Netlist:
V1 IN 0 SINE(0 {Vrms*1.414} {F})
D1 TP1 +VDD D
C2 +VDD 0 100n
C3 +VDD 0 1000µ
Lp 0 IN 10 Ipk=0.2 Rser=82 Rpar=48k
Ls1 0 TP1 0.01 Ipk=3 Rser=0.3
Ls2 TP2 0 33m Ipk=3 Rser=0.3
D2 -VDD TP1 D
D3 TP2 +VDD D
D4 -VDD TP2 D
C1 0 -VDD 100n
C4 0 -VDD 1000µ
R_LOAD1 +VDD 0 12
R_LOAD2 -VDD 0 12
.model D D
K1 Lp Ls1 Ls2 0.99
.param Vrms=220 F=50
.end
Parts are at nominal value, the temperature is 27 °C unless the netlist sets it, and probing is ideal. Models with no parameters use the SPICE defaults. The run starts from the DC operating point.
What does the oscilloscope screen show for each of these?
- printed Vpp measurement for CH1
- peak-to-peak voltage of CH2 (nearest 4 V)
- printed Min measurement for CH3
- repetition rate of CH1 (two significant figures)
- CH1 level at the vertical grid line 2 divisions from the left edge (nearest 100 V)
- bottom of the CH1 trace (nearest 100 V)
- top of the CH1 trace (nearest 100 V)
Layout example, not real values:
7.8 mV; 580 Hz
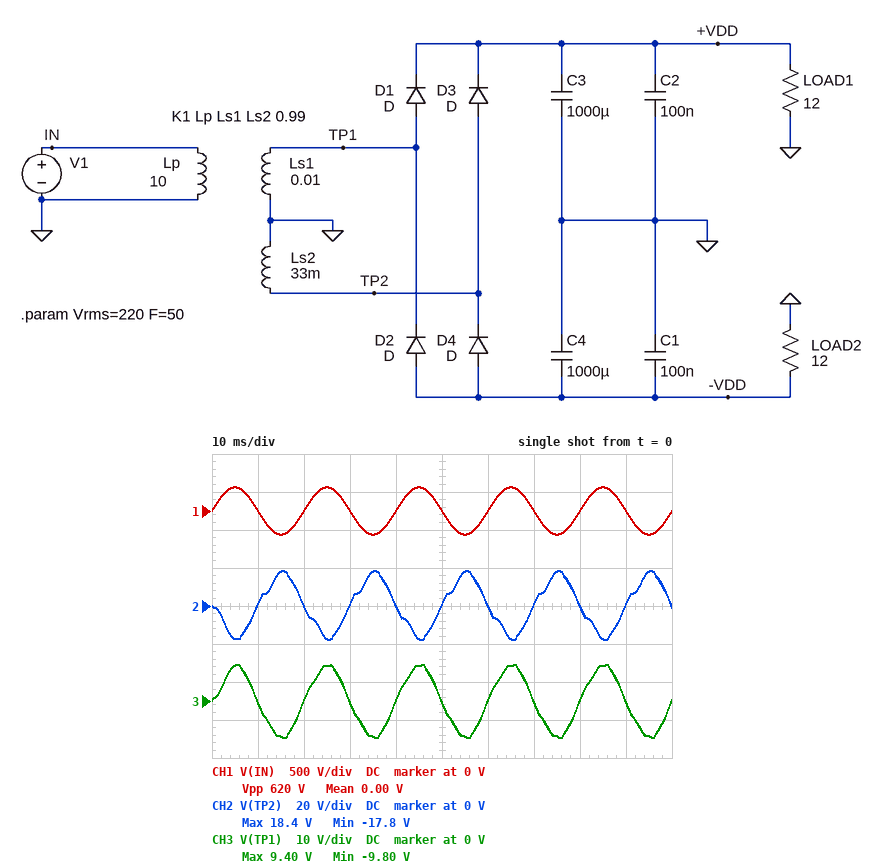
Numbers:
620 V; 36 V; -9.80 V; 50 Hz; 0 V; -300 V; 300 V
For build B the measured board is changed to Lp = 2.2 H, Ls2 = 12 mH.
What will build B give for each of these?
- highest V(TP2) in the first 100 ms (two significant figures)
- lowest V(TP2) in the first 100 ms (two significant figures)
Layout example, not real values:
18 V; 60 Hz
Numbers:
22 V; -20 V
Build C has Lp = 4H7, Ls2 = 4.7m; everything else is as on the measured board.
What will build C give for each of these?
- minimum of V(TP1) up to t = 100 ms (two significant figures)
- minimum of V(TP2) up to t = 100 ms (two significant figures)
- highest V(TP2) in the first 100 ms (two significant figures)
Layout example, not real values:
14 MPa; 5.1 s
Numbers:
-14 V; -9.2 V; 9.7 V
